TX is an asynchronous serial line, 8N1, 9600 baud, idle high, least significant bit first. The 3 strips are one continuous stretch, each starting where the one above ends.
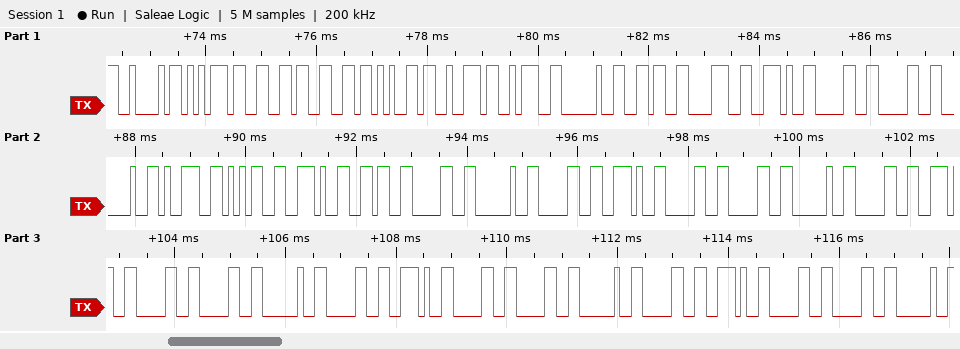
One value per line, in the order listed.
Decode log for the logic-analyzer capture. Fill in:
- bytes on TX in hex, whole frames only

42 75 66 66 65 72 3A 20 36 38 2E 30 30 20 39 35 2E 36 30 20 30 2E 30 30 20 30 2E 30 30 20 30 2E 30 30 20 30 2E 30 30 20
